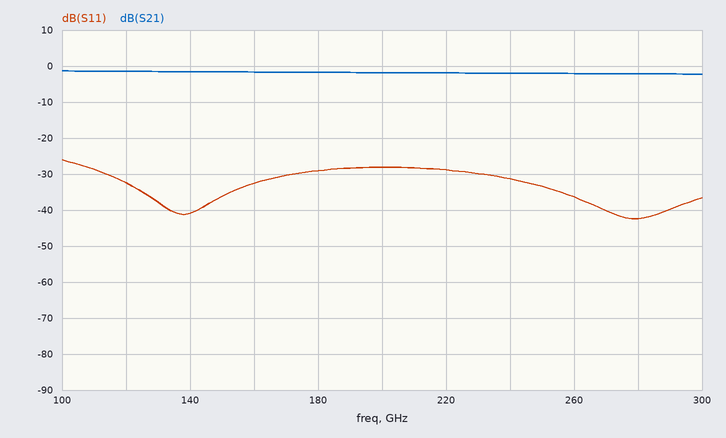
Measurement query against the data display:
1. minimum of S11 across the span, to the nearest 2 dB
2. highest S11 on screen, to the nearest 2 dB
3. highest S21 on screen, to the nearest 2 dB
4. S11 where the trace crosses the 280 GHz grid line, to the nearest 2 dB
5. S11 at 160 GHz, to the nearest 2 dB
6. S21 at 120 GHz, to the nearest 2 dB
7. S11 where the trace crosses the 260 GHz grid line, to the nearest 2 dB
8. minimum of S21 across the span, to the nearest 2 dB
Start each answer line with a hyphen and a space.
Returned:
- -42 dB
- -26 dB
- -2 dB
- -42 dB
- -32 dB
- -2 dB
- -36 dB
- -2 dB
